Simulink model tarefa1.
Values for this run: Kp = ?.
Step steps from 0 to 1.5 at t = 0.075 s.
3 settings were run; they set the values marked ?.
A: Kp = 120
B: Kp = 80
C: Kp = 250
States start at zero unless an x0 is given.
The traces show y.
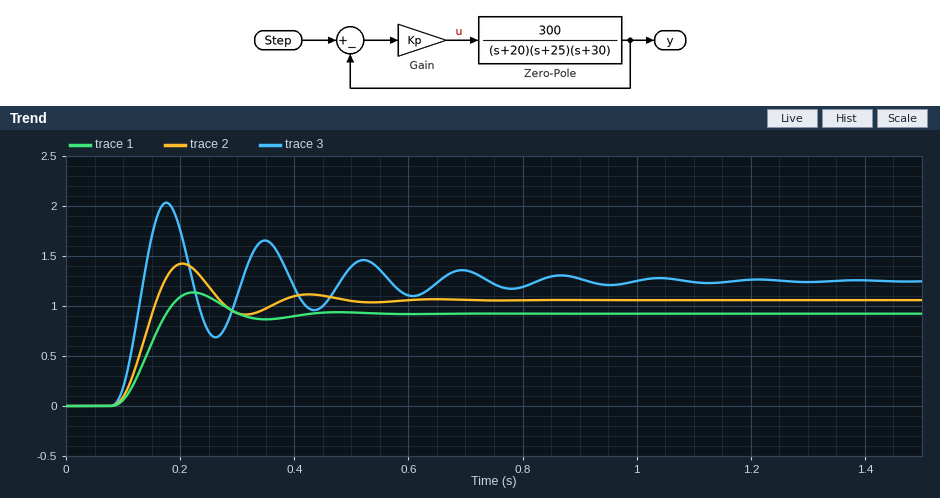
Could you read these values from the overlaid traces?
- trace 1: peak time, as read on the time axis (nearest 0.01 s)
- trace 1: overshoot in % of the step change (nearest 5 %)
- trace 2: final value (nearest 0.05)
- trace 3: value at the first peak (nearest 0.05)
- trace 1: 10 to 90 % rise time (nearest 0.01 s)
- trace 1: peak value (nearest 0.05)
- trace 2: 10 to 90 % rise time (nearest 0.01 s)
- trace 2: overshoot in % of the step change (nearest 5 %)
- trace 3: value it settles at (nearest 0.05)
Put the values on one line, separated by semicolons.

0.22 s; 25 %; 1.05; 2.05; 0.06 s; 1.15; 0.05 s; 35 %; 1.25
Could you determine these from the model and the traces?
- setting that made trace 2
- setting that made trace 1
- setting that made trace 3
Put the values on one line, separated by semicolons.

A; B; C
